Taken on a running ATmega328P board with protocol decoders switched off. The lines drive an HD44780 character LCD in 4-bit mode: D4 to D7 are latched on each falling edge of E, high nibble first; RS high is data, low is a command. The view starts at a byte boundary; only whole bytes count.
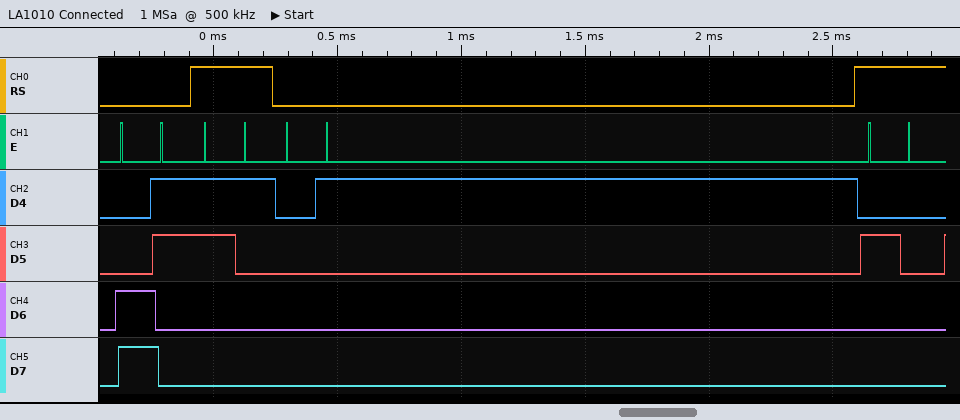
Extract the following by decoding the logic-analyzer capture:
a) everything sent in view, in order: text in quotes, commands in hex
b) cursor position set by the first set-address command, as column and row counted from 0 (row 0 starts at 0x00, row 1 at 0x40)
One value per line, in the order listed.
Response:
0xC3 "1" 0x01 " "
column 3, row 1
